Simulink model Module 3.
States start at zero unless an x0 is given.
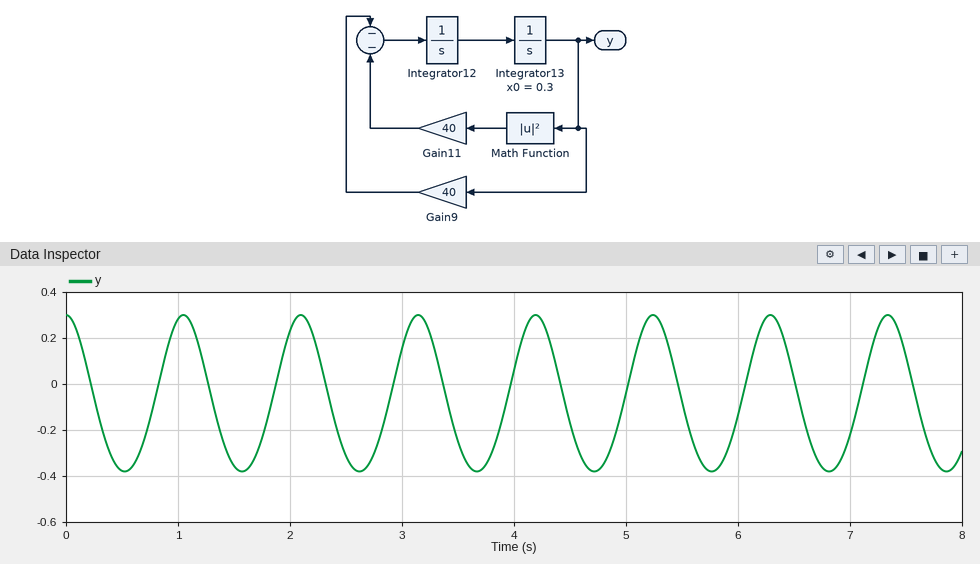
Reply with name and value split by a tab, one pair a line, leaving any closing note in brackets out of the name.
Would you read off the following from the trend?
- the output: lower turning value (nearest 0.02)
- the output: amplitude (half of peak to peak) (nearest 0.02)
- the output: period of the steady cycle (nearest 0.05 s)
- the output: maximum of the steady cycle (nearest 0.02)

the output: lower turning value	-0.38
the output: amplitude (half of peak to peak)	0.34
the output: period of the steady cycle	1.05 s
the output: maximum of the steady cycle	0.30
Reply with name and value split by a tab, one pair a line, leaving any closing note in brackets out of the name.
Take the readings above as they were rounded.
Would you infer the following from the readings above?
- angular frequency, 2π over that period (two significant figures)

angular frequency, 2π over that period	6.0 rad/s
